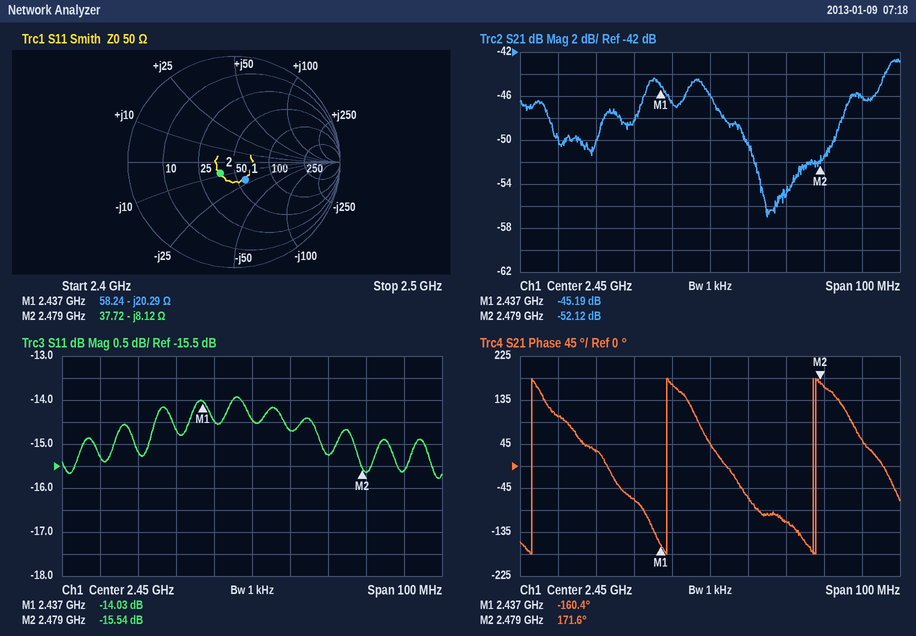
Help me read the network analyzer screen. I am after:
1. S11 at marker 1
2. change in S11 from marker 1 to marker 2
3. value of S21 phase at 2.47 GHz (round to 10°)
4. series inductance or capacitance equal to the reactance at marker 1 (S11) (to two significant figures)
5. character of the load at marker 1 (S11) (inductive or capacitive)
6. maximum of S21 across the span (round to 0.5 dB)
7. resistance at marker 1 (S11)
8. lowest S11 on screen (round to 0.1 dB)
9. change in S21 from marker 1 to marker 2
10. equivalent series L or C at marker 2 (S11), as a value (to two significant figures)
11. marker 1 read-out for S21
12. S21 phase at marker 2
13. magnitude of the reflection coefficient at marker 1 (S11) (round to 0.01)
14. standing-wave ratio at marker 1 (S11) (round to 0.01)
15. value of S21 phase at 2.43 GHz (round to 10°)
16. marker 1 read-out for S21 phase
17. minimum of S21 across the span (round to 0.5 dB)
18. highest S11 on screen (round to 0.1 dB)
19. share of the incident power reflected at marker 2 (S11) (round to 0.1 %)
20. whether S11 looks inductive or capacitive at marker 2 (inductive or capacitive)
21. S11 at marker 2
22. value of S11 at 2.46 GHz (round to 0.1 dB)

-14.03 dB
-1.51 dB
-110°
3.2 pF
capacitive
-42.5 dB
58.24 Ω
-15.8 dB
-6.93 dB
7.9 pF
-45.19 dB
171.6°
0.20
1.50
-70°
-160.4°
-57.0 dB
-13.9 dB
2.8 %
capacitive
-15.54 dB
-14.7 dB
